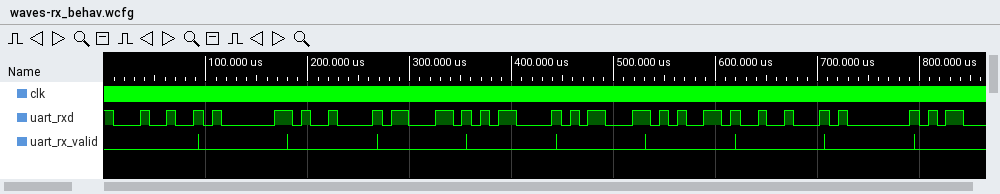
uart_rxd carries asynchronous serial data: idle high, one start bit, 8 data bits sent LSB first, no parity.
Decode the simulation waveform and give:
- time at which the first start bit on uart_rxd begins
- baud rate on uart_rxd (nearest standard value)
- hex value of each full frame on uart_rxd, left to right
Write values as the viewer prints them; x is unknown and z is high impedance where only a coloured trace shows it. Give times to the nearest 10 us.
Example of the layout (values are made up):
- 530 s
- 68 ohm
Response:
- 10 us
- 115200 baud
- 24, 81, 09, 63, 0D, 8D, 65, 12, 01
